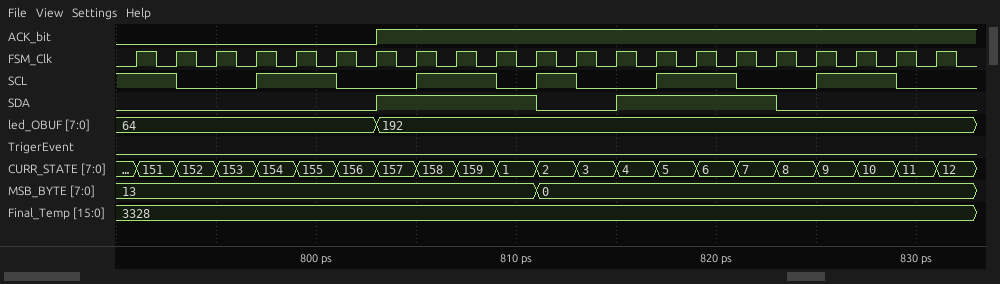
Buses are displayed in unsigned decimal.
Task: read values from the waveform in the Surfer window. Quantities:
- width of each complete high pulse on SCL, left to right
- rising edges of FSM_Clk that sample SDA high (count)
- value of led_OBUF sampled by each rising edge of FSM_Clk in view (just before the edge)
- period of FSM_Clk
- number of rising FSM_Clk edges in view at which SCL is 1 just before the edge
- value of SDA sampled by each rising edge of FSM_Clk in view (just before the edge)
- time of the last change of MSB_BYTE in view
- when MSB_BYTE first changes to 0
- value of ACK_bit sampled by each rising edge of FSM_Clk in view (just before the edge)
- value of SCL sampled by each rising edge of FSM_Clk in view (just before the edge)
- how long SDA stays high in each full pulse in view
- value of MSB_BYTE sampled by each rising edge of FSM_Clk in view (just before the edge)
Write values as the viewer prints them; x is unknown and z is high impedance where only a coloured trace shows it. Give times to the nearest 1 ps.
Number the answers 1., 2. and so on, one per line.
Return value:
1. 4 ps, 4 ps, 2 ps, 4 ps, 4 ps
2. 8
3. 64, 64, 64, 64, 64, 64, 64, 192, 192, 192, 192, 192, 192, 192, 192, 192, 192, 192, 192, 192, 192
4. 2 ps
5. 11
6. 0 0 0 0 0 0 0 1 1 1 1 0 0 1 1 1 1 0 0 0 0
7. 811 ps
8. 811 ps
9. 0 0 0 0 0 0 0 1 1 1 1 1 1 1 1 1 1 1 1 1 1
10. 1 1 0 0 1 1 0 0 1 1 0 1 0 0 1 1 0 0 1 1 0
11. 8 ps, 8 ps
12. 13, 13, 13, 13, 13, 13, 13, 13, 13, 13, 13, 0, 0, 0, 0, 0, 0, 0, 0, 0, 0
